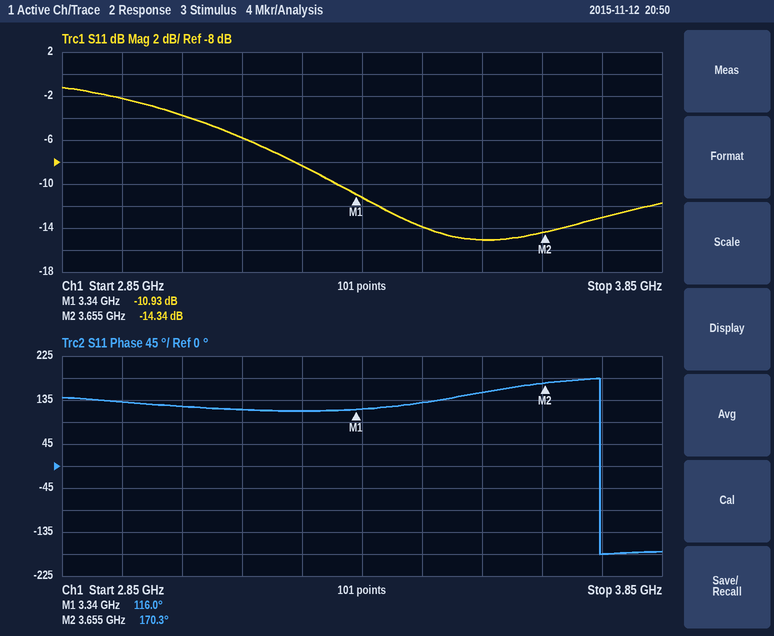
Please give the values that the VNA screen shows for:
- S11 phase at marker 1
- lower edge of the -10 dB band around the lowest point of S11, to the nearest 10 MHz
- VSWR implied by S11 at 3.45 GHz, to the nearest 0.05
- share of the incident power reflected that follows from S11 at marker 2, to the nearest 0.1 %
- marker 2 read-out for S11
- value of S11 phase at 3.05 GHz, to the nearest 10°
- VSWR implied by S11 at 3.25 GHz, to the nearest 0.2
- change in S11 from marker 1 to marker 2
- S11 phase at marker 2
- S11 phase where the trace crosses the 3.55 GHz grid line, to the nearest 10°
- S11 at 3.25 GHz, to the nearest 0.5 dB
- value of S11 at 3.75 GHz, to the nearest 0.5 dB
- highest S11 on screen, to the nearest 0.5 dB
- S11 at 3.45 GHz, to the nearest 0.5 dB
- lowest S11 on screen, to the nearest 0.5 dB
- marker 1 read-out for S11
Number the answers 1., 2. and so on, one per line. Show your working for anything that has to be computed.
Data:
1. 116.0°
2. 3.31 GHz
3. |Γ| = 10^(-14/20) = 0.1995; VSWR = (1 + 0.1995)/(1 − 0.1995) ≈ 1.50
4. 10^(-14.34/10) ≈ 3.7 %
5. -14.34 dB
6. 120°
7. |Γ| = 10^(-8.5/20) = 0.3758; VSWR = (1 + 0.3758)/(1 − 0.3758) ≈ 2.2
8. -14.34 − (-10.93) = -3.41 dB
9. 170.3°
10. 150°
11. -8.5 dB
12. -13.0 dB
13. -1.0 dB
14. -14.0 dB
15. -15.0 dB
16. -10.93 dB
